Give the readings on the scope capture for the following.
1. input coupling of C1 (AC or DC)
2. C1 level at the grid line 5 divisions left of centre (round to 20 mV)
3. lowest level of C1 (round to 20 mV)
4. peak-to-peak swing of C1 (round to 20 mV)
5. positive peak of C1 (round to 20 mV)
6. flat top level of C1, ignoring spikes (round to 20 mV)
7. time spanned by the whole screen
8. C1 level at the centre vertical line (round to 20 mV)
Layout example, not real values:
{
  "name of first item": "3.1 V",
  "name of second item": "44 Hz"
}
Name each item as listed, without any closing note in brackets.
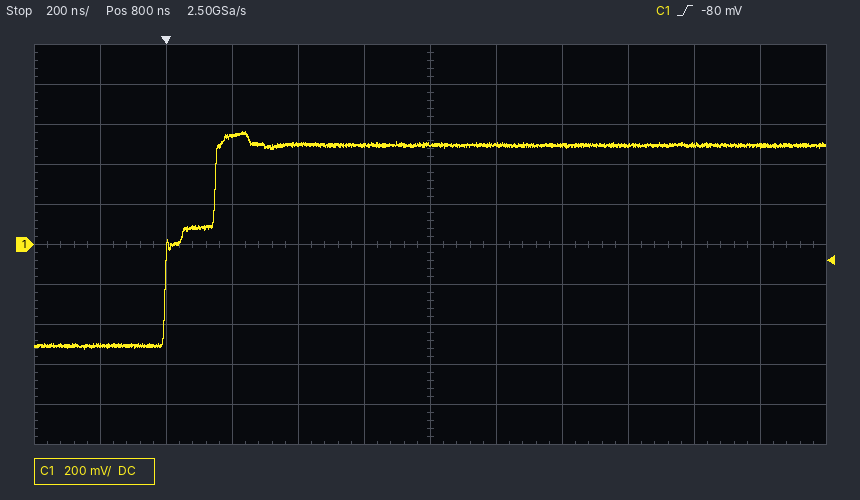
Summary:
{
  "input coupling of C1": "DC",
  "C1 level at the grid line 5 divisions left of centre": "-500 mV",
  "lowest level of C1": "-520 mV",
  "peak-to-peak swing of C1": "1.08 V",
  "positive peak of C1": "560 mV",
  "flat top level of C1, ignoring spikes": "500 mV",
  "time spanned by the whole screen": "2.4 µs",
  "C1 level at the centre vertical line": "500 mV"
}
